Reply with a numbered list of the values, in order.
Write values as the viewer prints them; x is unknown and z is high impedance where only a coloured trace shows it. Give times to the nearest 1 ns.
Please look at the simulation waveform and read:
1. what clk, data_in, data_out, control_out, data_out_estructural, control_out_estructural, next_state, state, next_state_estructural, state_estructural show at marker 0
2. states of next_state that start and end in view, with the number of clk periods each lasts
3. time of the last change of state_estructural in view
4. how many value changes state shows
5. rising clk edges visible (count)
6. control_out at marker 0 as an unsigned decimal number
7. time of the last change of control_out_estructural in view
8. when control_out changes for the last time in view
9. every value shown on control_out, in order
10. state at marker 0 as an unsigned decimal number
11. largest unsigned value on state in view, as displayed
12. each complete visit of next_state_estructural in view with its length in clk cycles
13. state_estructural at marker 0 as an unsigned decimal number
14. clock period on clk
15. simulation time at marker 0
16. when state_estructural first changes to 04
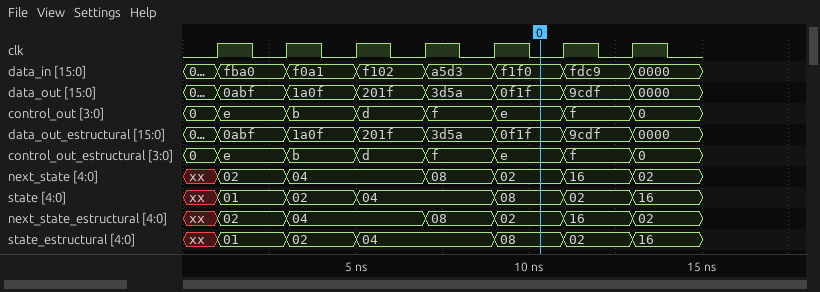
1. clk=0, data_in=f1f0, data_out=0f1f, control_out=e, data_out_estructural=0f1f, control_out_estructural=e, next_state=02, state=08, next_state_estructural=02, state_estructural=08
2. 02: 1, 04: 2, 08: 1, 02: 1, 16: 1
3. 13 ns
4. 6
5. 7
6. 14
7. 13 ns
8. 13 ns
9. 0, e, b, d, f, e, f, 0
10. 8
11. 16
12. 02: 1, 04: 2, 08: 1, 02: 1, 16: 1
13. 8
14. 2 ns
15. 10 ns
16. 5 ns
